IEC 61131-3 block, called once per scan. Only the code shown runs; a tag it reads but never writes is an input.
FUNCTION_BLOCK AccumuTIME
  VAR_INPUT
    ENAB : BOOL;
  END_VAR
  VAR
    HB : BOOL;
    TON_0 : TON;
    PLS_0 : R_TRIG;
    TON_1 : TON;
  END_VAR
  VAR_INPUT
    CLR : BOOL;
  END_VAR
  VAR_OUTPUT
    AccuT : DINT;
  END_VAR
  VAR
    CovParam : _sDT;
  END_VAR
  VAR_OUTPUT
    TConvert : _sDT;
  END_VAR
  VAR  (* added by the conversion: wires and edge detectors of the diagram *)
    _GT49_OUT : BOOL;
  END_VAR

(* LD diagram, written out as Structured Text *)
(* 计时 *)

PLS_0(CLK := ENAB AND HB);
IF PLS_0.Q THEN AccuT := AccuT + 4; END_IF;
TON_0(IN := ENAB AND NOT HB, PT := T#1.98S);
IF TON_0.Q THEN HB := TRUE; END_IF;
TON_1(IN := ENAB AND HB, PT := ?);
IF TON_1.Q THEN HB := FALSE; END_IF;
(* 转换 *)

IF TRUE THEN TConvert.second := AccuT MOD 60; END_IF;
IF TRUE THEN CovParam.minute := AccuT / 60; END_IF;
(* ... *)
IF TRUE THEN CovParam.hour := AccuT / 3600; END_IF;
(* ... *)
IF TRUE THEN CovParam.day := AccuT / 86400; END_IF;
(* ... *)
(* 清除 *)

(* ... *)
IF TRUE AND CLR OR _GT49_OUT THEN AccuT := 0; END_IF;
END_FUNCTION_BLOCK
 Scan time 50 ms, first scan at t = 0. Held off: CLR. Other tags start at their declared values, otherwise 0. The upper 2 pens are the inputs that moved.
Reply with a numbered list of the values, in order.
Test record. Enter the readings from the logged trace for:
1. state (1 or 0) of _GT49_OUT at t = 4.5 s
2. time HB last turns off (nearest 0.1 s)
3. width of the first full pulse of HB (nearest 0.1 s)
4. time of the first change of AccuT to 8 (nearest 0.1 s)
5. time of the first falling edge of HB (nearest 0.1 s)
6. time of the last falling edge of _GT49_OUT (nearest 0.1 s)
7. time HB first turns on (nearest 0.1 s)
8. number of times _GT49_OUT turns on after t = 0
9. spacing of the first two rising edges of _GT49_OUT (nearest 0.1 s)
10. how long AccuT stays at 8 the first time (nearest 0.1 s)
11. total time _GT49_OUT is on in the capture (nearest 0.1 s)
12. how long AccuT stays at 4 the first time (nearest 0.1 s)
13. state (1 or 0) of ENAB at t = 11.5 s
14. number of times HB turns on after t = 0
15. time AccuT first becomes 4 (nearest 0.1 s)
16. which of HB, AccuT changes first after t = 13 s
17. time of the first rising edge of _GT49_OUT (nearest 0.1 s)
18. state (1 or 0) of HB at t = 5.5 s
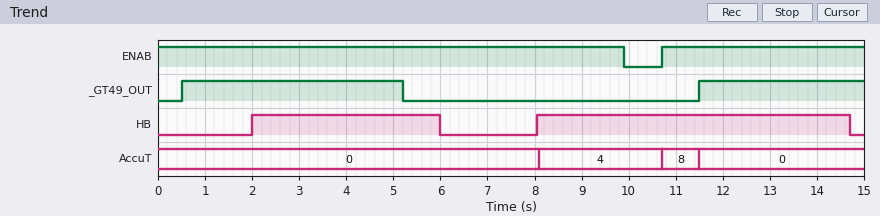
1. 1
2. 14.7 s
3. 4.0 s
4. 10.7 s
5. 6.0 s
6. 5.2 s
7. 2.0 s
8. 2
9. 11.0 s
10. 0.8 s
11. 8.2 s
12. 2.6 s
13. 1
14. 2
15. 8.1 s
16. HB
17. 0.5 s
18. 1
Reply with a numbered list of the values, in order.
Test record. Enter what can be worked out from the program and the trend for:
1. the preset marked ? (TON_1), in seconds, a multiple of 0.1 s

1. 4.0 s
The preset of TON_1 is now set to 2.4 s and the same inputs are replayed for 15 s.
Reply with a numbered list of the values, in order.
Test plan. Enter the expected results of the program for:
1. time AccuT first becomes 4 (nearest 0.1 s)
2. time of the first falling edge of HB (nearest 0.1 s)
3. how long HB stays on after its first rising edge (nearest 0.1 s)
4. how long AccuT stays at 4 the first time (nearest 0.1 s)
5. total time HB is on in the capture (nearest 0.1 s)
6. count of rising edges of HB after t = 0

1. 6.5 s
2. 4.4 s
3. 2.4 s
4. 5.0 s
5. 7.1 s
6. 3
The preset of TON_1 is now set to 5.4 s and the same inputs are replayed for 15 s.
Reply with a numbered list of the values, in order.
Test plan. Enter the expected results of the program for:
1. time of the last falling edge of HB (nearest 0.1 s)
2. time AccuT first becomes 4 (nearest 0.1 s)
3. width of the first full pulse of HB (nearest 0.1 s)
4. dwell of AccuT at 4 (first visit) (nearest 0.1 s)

1. 7.4 s
2. 9.5 s
3. 5.4 s
4. 1.2 s
